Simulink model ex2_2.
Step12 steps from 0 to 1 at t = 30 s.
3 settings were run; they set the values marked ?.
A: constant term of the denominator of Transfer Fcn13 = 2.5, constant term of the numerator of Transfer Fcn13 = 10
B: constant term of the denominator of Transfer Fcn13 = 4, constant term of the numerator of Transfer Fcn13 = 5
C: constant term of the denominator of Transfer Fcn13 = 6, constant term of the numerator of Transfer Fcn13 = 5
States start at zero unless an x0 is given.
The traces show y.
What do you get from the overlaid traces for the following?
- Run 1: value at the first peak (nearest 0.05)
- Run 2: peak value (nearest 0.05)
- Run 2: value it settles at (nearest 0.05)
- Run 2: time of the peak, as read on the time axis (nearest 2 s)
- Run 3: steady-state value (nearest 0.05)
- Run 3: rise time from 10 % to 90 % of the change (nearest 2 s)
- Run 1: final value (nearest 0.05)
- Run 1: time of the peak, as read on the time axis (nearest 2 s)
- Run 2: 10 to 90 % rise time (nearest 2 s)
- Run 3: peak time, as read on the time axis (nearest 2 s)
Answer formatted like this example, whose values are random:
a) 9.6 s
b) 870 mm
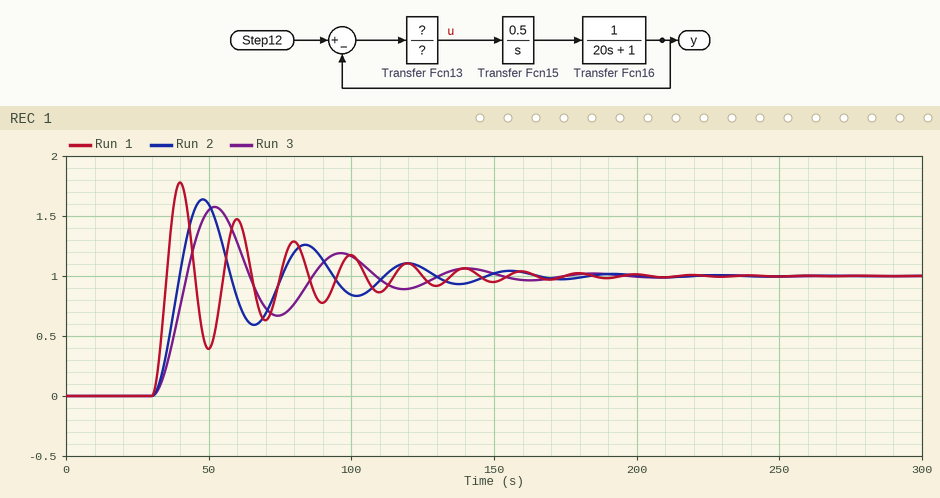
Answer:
a) 1.80
b) 1.65
c) 1.00
d) 48 s
e) 1.00
f) 8 s
g) 1.00
h) 40 s
i) 6 s
j) 52 s
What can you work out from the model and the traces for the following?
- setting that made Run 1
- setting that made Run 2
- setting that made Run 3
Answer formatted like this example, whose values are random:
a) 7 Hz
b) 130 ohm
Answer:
a) A
b) B
c) C
